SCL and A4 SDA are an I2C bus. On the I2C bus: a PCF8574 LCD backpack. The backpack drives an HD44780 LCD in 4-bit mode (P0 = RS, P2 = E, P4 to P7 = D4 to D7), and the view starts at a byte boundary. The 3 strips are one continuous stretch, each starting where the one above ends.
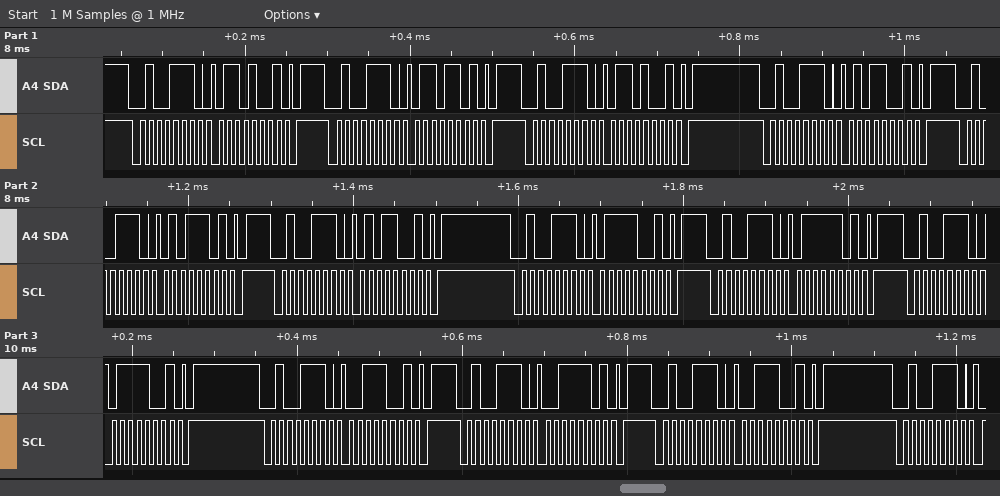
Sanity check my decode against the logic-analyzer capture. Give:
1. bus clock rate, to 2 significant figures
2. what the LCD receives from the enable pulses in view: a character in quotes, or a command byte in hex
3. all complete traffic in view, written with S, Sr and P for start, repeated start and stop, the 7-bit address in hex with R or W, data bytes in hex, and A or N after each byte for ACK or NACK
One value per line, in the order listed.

100 kHz
'e' 's'
S 27W A 69 A P S 27W A 6D A P S 27W A 69 A P S 27W A 59 A P S 27W A 5D A P S 27W A 59 A P S 27W A 79 A P S 27W A 7D A P S 27W A 79 A P S 27W A 39 A P S 27W A 3D A P S 27W A 39 A P S 27W A
